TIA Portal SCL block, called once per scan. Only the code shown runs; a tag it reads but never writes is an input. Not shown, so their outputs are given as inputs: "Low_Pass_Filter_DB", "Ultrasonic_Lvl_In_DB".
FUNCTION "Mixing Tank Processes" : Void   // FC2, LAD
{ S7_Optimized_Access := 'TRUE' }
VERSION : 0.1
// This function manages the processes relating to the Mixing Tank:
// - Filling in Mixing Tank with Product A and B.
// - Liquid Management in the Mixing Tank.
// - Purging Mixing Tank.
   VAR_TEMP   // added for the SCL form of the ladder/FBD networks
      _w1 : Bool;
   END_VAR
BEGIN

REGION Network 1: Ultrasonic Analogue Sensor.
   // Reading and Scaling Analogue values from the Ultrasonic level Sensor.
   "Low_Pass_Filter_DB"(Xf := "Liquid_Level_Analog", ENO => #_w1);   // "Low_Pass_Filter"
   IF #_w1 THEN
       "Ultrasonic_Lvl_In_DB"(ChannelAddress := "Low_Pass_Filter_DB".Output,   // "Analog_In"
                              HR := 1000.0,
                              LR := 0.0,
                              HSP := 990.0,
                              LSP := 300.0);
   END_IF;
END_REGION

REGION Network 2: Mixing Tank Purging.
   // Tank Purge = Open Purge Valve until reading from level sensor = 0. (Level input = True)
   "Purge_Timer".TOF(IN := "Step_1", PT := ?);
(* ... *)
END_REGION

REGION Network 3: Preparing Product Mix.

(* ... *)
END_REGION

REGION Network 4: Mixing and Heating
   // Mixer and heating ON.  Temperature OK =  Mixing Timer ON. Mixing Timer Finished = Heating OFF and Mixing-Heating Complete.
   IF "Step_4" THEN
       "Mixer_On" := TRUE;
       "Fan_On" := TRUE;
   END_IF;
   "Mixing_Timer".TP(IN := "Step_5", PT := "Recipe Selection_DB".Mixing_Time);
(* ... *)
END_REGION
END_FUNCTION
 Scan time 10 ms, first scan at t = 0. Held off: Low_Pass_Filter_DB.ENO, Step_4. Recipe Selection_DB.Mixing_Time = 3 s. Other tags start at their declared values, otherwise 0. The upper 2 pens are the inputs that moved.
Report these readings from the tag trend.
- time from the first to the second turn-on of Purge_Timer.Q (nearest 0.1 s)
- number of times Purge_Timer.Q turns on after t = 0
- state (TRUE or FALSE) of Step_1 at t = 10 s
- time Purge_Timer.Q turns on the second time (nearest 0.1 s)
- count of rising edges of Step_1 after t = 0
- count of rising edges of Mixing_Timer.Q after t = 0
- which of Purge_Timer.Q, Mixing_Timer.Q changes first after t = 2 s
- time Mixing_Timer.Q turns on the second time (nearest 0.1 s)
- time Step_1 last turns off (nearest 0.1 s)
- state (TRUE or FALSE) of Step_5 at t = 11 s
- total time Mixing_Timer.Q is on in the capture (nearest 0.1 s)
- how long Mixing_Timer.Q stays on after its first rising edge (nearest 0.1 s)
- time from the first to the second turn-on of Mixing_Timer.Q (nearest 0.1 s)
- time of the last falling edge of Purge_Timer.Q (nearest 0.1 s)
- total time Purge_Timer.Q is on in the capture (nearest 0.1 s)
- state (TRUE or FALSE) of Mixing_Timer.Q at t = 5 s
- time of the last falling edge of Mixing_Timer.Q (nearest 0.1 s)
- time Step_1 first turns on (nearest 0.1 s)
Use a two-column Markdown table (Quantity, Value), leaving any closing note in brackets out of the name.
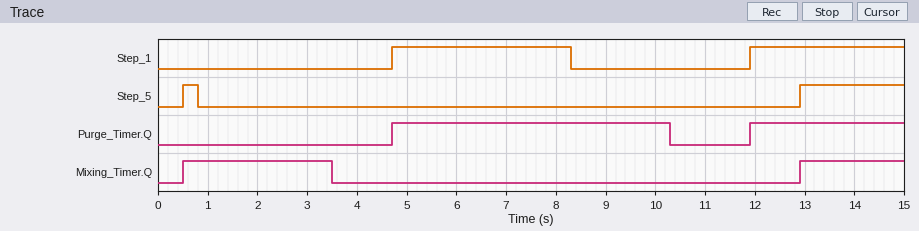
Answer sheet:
| Quantity | Value |
|---|---|
| time from the first to the second turn-on of Purge_Timer.Q | 7.2 s |
| number of times Purge_Timer.Q turns on after t = 0 | 2 |
| state (TRUE or FALSE) of Step_1 at t = 10 s | FALSE |
| time Purge_Timer.Q turns on the second time | 11.9 s |
| count of rising edges of Step_1 after t = 0 | 2 |
| count of rising edges of Mixing_Timer.Q after t = 0 | 2 |
| which of Purge_Timer.Q, Mixing_Timer.Q changes first after t = 2 s | Mixing_Timer.Q |
| time Mixing_Timer.Q turns on the second time | 12.9 s |
| time Step_1 last turns off | 8.3 s |
| state (TRUE or FALSE) of Step_5 at t = 11 s | FALSE |
| total time Mixing_Timer.Q is on in the capture | 5.1 s |
| how long Mixing_Timer.Q stays on after its first rising edge | 3.0 s |
| time from the first to the second turn-on of Mixing_Timer.Q | 12.4 s |
| time of the last falling edge of Purge_Timer.Q | 10.3 s |
| total time Purge_Timer.Q is on in the capture | 8.7 s |
| state (TRUE or FALSE) of Mixing_Timer.Q at t = 5 s | FALSE |
| time of the last falling edge of Mixing_Timer.Q | 3.5 s |
| time Step_1 first turns on | 4.7 s |
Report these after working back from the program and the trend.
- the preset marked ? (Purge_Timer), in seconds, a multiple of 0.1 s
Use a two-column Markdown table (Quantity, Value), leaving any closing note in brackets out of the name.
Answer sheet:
| Quantity | Value |
|---|---|
| the preset marked ? (Purge_Timer), in seconds, a multiple of 0.1 s | 2.0 s |
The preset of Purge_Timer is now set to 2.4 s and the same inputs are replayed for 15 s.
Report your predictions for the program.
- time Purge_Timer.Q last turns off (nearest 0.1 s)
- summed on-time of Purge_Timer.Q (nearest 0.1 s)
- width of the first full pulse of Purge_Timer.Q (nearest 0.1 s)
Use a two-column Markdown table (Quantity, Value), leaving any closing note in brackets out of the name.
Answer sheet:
| Quantity | Value |
|---|---|
| time Purge_Timer.Q last turns off | 10.7 s |
| summed on-time of Purge_Timer.Q | 9.1 s |
| width of the first full pulse of Purge_Timer.Q | 6.0 s |
